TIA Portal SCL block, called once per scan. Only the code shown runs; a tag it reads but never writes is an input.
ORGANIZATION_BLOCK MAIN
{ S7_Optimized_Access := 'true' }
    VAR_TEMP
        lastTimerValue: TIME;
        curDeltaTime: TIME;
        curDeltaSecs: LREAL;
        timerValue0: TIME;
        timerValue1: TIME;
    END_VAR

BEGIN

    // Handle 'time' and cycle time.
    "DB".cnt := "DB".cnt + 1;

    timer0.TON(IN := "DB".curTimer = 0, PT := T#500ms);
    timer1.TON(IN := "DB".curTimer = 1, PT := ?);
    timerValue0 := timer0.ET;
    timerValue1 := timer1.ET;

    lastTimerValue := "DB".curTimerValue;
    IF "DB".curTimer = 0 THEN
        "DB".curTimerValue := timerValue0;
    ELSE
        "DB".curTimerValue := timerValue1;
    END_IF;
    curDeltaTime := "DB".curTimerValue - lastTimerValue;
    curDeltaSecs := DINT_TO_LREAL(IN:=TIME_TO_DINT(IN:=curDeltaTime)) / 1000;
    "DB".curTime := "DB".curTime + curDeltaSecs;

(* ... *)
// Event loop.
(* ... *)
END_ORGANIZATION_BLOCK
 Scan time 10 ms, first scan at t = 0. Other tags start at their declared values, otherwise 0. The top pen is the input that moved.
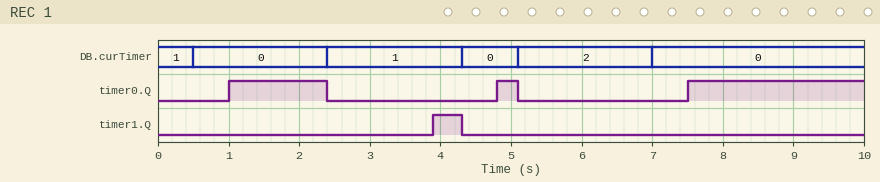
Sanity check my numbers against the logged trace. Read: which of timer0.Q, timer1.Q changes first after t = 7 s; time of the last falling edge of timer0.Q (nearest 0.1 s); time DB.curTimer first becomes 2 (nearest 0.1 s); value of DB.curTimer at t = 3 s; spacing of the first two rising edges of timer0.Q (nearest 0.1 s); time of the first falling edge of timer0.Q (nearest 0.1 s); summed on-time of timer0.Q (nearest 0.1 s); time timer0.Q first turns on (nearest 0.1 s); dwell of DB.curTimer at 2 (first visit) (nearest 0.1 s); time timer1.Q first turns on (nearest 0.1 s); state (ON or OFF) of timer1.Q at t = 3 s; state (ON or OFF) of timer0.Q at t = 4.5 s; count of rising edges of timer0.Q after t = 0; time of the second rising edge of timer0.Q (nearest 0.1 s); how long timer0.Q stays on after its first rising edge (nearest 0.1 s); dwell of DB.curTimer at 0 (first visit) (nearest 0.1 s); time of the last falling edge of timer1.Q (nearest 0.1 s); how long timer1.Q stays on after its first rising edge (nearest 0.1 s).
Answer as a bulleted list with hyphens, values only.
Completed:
- timer0.Q
- 5.1 s
- 5.1 s
- 1
- 3.8 s
- 2.4 s
- 4.2 s
- 1.0 s
- 1.9 s
- 3.9 s
- OFF
- OFF
- 3
- 4.8 s
- 1.4 s
- 1.9 s
- 4.3 s
- 0.4 s
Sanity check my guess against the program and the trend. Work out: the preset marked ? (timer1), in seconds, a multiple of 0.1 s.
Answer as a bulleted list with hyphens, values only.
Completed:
- 1.5 s
